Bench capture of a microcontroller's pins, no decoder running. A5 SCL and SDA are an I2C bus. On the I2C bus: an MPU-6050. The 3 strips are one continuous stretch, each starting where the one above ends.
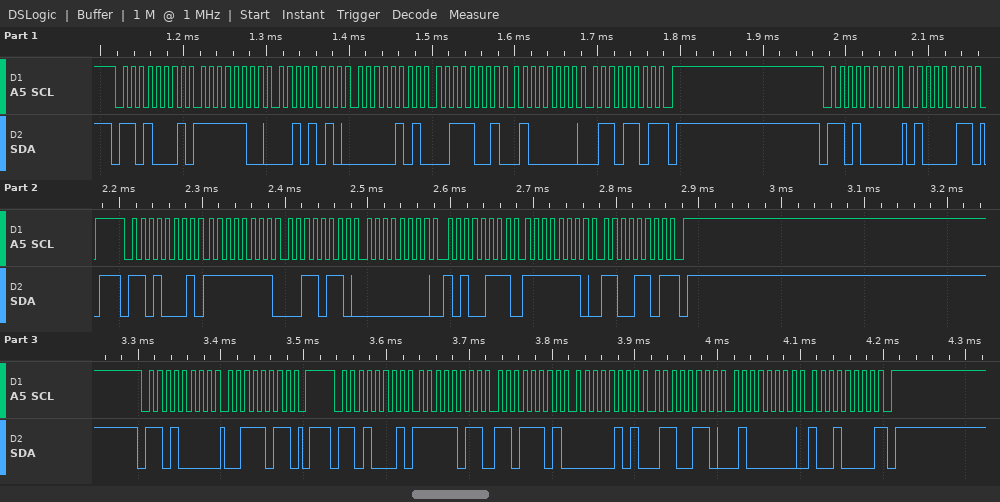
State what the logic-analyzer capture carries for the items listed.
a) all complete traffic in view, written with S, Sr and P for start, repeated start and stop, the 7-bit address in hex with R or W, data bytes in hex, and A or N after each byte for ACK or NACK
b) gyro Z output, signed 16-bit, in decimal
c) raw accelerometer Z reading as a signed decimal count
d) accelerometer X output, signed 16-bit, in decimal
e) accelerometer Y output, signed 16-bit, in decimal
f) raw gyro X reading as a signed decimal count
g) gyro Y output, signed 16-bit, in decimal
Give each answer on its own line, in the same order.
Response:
S 68R A FC A 2A A 05 A 39 A 40 A 6D N P S 68W A 43 A P S 68R A FF A 36 A 00 A A7 A FE A CD N P S 68W A 3B A P S 68R A FB A DD A 05 A 66 A 40 A 90 N P
-307
16528
-1059
1382
-202
167
